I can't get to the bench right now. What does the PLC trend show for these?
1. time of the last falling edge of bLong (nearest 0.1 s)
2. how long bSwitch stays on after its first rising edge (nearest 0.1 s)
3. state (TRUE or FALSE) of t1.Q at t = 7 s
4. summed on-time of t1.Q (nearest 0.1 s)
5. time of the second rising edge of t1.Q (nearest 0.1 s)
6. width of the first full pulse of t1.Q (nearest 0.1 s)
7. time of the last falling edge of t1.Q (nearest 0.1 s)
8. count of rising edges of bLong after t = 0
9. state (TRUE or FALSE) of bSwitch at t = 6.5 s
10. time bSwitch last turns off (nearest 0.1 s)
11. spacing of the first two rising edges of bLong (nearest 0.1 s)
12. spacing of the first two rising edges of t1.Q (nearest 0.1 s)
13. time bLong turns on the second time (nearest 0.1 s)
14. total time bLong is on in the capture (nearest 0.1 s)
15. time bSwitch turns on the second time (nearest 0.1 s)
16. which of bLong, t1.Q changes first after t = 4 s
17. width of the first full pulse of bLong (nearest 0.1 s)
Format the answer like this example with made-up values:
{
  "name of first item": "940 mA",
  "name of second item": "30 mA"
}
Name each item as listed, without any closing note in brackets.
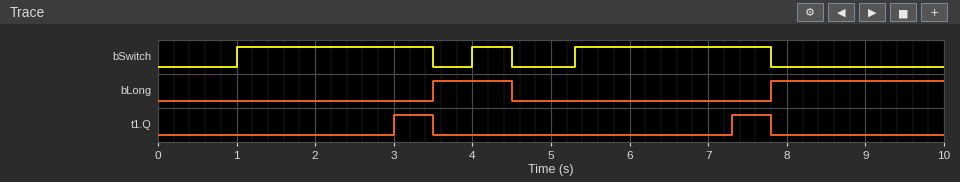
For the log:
{
  "time of the last falling edge of bLong": "4.5 s",
  "how long bSwitch stays on after its first rising edge": "2.5 s",
  "state (TRUE or FALSE) of t1.Q at t = 7 s": "FALSE",
  "summed on-time of t1.Q": "1.0 s",
  "time of the second rising edge of t1.Q": "7.3 s",
  "width of the first full pulse of t1.Q": "0.5 s",
  "time of the last falling edge of t1.Q": "7.8 s",
  "count of rising edges of bLong after t = 0": "2",
  "state (TRUE or FALSE) of bSwitch at t = 6.5 s": "TRUE",
  "time bSwitch last turns off": "7.8 s",
  "spacing of the first two rising edges of bLong": "4.3 s",
  "spacing of the first two rising edges of t1.Q": "4.3 s",
  "time bLong turns on the second time": "7.8 s",
  "total time bLong is on in the capture": "3.2 s",
  "time bSwitch turns on the second time": "4.0 s",
  "which of bLong, t1.Q changes first after t = 4 s": "bLong",
  "width of the first full pulse of bLong": "1.0 s"
}
